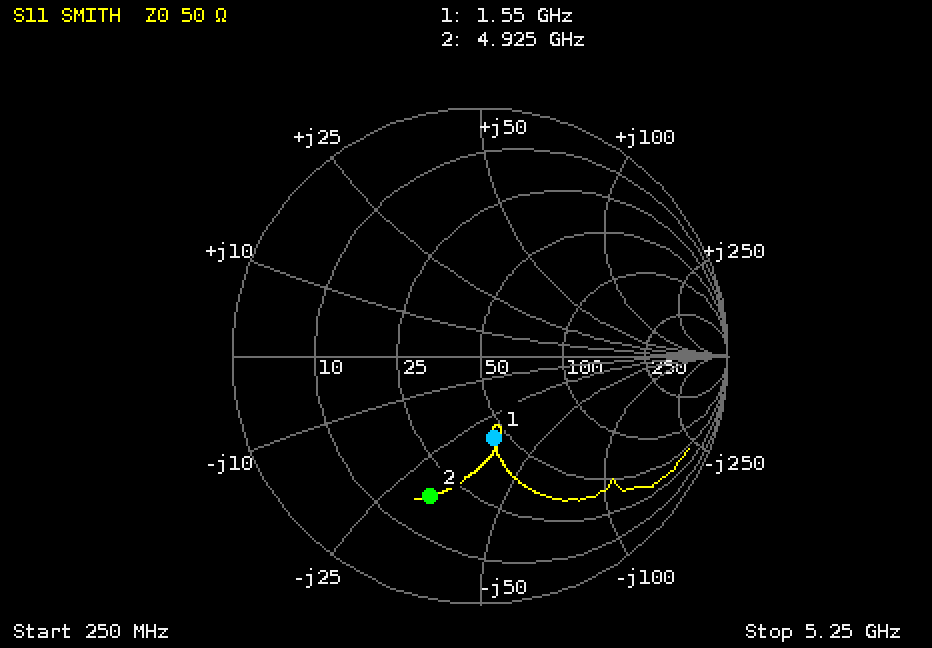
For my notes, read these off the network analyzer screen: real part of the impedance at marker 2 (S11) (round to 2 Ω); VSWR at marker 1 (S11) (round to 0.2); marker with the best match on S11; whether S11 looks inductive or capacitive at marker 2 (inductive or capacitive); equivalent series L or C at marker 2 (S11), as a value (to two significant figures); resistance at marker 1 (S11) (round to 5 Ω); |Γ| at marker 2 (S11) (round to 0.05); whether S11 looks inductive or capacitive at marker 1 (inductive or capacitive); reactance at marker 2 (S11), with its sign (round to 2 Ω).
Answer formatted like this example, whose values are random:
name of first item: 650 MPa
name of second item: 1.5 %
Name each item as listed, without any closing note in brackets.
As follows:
real part of the impedance at marker 2 (S11): 18 Ω
VSWR at marker 1 (S11): 2.0
marker with the best match on S11: marker 1
whether S11 looks inductive or capacitive at marker 2: capacitive
equivalent series L or C at marker 2 (S11), as a value: 1.0 pF
resistance at marker 1 (S11): 45 Ω
|Γ| at marker 2 (S11): 0.60
whether S11 looks inductive or capacitive at marker 1: capacitive
reactance at marker 2 (S11), with its sign: -32 Ω
